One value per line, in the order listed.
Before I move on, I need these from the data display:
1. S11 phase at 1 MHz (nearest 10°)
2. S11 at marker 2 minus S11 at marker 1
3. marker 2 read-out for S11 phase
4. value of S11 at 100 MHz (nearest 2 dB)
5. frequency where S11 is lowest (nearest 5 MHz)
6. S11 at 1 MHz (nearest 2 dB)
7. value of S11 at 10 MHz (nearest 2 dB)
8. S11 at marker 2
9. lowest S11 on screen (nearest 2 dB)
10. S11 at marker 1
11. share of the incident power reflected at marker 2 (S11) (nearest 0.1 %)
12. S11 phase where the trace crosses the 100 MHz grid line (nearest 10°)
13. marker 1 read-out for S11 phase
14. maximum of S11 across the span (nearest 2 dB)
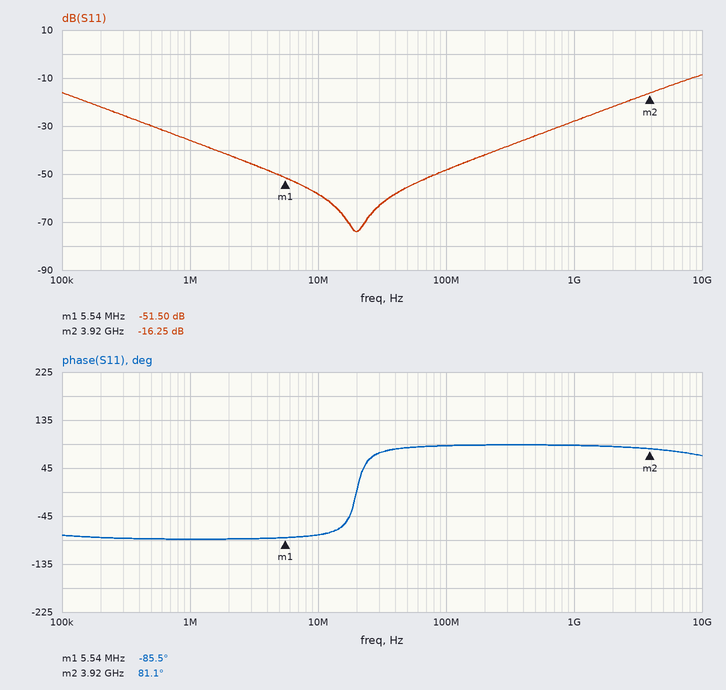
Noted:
-90°
35.25 dB
81.1°
-48 dB
20 MHz
-36 dB
-58 dB
-16.25 dB
-74 dB
-51.50 dB
2.4 %
90°
-85.5°
-8 dB
